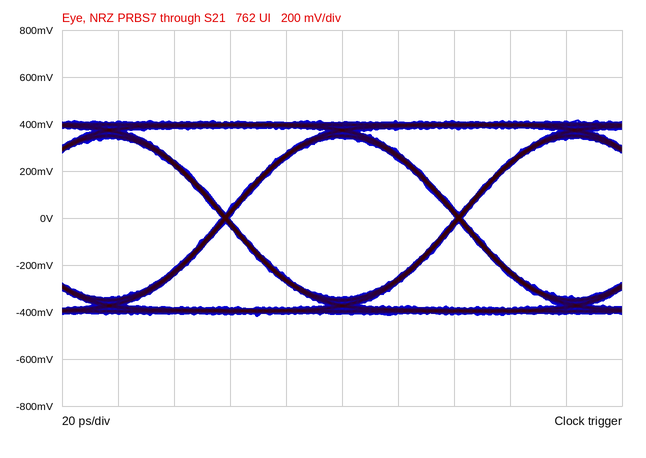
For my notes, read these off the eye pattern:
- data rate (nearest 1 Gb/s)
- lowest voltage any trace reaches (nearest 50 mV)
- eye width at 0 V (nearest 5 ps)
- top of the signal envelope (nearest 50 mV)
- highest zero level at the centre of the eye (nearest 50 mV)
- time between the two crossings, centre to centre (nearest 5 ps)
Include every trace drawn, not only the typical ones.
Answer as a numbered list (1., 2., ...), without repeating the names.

1. 12 Gb/s
2. -400 mV
3. 80 ps
4. 400 mV
5. -350 mV
6. 85 ps
